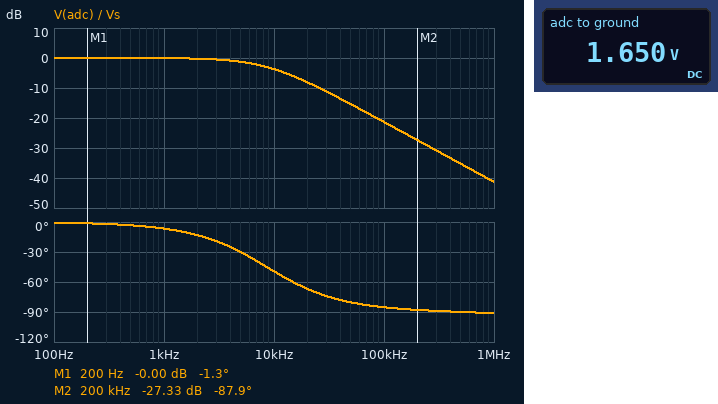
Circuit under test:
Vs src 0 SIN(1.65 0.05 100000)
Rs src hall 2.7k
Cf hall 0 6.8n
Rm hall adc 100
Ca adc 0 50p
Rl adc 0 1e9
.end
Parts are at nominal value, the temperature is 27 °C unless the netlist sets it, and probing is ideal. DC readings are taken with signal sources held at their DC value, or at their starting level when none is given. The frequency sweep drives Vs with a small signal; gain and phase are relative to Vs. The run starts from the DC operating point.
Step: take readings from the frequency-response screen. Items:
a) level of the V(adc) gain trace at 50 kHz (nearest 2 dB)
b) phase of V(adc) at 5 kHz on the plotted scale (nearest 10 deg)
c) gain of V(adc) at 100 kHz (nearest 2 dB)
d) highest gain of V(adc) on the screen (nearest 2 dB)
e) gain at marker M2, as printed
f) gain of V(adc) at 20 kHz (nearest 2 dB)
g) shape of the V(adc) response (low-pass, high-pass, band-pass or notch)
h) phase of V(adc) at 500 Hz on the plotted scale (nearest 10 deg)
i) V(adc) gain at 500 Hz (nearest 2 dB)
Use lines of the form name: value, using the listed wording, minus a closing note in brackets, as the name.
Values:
level of the V(adc) gain trace at 50 kHz: -16 dB
phase of V(adc) at 5 kHz on the plotted scale: -30 deg
gain of V(adc) at 100 kHz: -22 dB
highest gain of V(adc) on the screen: 0 dB
gain at marker M2, as printed: -27.33 dB
gain of V(adc) at 20 kHz: -8 dB
shape of the V(adc) response: low-pass
phase of V(adc) at 500 Hz on the plotted scale: 0 deg
V(adc) gain at 500 Hz: 0 dB
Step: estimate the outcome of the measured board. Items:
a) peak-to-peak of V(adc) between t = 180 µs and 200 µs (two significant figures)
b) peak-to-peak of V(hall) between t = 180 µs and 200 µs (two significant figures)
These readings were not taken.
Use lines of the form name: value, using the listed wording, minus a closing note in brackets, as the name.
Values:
peak-to-peak of V(adc) between t = 180 µs and 200 µs: 8.6 mV
peak-to-peak of V(hall) between t = 180 µs and 200 µs: 8.6 mV
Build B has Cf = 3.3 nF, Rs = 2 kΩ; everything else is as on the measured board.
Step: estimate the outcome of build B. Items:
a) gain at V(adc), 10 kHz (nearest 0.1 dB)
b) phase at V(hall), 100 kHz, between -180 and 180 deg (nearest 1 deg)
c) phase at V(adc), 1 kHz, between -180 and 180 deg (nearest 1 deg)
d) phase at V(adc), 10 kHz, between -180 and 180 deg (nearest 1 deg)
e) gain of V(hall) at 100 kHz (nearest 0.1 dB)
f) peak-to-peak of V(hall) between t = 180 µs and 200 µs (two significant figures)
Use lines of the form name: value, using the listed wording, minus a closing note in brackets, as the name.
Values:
gain at V(adc), 10 kHz: -0.7 dB
phase at V(hall), 100 kHz, between -180 and 180 deg: -77 deg
phase at V(adc), 1 kHz, between -180 and 180 deg: -2 deg
phase at V(adc), 10 kHz, between -180 and 180 deg: -23 deg
gain of V(hall) at 100 kHz: -12.7 dB
peak-to-peak of V(hall) between t = 180 µs and 200 µs: 23 mV
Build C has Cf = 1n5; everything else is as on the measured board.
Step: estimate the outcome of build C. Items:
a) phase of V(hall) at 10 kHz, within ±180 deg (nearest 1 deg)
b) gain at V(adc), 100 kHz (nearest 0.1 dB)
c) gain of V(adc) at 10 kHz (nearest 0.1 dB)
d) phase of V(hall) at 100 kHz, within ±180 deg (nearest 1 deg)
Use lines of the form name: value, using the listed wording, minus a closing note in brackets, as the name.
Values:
phase of V(hall) at 10 kHz, within ±180 deg: -15 deg
gain at V(adc), 100 kHz: -9.0 dB
gain of V(adc) at 10 kHz: -0.3 dB
phase of V(hall) at 100 kHz, within ±180 deg: -69 deg
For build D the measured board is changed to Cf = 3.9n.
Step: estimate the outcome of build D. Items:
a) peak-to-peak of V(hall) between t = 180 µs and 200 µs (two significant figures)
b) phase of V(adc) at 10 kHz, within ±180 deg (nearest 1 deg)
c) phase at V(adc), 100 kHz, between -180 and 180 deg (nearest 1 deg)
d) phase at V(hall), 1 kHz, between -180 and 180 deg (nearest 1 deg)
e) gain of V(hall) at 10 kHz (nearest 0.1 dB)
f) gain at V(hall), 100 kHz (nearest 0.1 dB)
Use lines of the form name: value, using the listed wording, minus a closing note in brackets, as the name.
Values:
peak-to-peak of V(hall) between t = 180 µs and 200 µs: 15 mV
phase of V(adc) at 10 kHz, within ±180 deg: -34 deg
phase at V(adc), 100 kHz, between -180 and 180 deg: -82 deg
phase at V(hall), 1 kHz, between -180 and 180 deg: -4 deg
gain of V(hall) at 10 kHz: -1.6 dB
gain at V(hall), 100 kHz: -16.6 dB
